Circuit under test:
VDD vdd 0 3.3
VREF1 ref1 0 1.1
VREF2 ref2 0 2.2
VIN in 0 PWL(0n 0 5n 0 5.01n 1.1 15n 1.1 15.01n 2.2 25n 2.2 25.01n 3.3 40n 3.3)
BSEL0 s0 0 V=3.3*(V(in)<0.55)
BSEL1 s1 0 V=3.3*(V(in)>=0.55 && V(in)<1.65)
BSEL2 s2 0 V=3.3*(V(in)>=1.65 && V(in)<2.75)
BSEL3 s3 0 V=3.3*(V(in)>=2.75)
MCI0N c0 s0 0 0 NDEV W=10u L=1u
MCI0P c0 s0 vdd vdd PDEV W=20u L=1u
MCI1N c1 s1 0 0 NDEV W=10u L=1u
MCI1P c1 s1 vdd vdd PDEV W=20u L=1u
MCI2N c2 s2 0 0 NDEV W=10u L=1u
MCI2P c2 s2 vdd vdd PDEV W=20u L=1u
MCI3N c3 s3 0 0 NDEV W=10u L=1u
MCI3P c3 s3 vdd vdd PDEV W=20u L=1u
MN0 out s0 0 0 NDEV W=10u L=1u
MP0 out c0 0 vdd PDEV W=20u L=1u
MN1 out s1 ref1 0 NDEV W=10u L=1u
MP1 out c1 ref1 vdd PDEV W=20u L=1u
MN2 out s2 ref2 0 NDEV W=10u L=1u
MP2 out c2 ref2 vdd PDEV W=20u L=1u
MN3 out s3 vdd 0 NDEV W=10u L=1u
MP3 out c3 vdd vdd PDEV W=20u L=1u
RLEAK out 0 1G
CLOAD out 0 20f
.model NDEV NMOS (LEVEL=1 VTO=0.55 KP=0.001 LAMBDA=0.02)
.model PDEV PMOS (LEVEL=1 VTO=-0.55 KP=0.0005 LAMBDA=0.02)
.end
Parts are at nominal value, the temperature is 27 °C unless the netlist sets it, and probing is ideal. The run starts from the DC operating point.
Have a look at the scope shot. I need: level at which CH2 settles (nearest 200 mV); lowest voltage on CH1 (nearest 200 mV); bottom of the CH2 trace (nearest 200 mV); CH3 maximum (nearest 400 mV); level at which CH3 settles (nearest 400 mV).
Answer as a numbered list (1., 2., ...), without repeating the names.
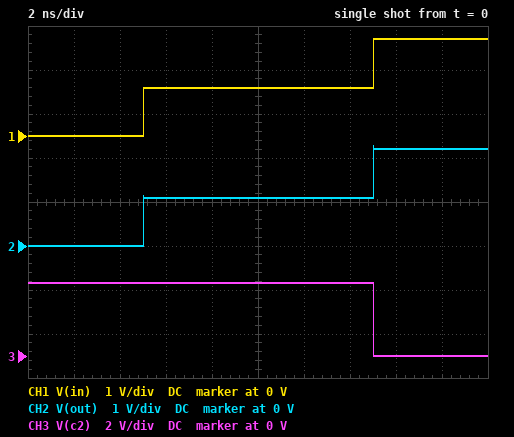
1. 2.2 V
2. 0 V
3. 0 V
4. 3.2 V
5. 0 V
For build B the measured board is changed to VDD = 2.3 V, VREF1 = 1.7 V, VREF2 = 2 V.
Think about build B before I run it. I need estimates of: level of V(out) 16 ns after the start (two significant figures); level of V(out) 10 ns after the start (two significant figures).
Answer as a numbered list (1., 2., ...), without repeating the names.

1. 2.0 V
2. 1.7 V
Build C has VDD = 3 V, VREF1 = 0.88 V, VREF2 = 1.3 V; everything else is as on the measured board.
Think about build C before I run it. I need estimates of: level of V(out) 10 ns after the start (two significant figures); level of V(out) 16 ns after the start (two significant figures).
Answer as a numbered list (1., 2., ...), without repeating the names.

1. 880 mV
2. 1.3 V
